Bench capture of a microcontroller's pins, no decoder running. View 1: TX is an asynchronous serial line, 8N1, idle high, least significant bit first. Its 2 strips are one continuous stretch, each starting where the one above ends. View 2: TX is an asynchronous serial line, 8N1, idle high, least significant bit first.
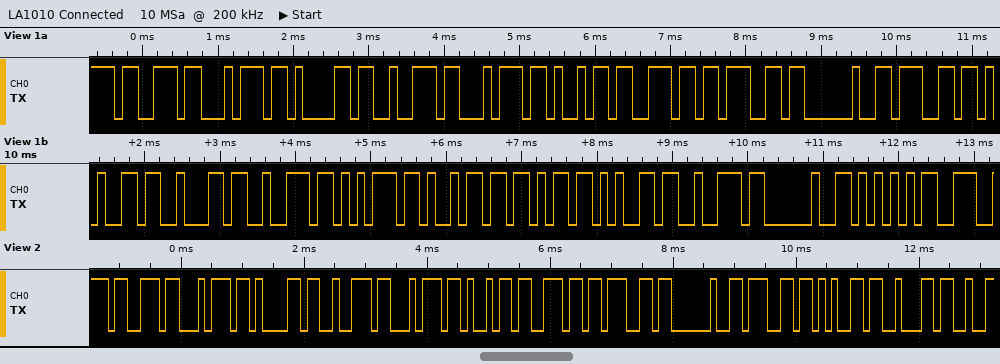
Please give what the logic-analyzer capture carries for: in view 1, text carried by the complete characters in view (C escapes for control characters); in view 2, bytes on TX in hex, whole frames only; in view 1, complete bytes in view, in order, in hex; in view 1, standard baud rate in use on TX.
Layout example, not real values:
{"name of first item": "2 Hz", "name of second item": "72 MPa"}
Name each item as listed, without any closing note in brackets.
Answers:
{"in view 1, text carried by the complete characters in view": "\"starting gebruiker U\"", "in view 2, bytes on TX in hex, whole frames only": "0x73 0x74 0x61 0x72 0x74 0x69 0x6E 0x67 0x20 0x67 0x65 0x62", "in view 1, complete bytes in view, in order, in hex": "73 74 61 72 74 69 6E 67 20 67 65 62 72 75 69 6B 65 72 20 55", "in view 1, standard baud rate in use on TX": "9600 baud"}
